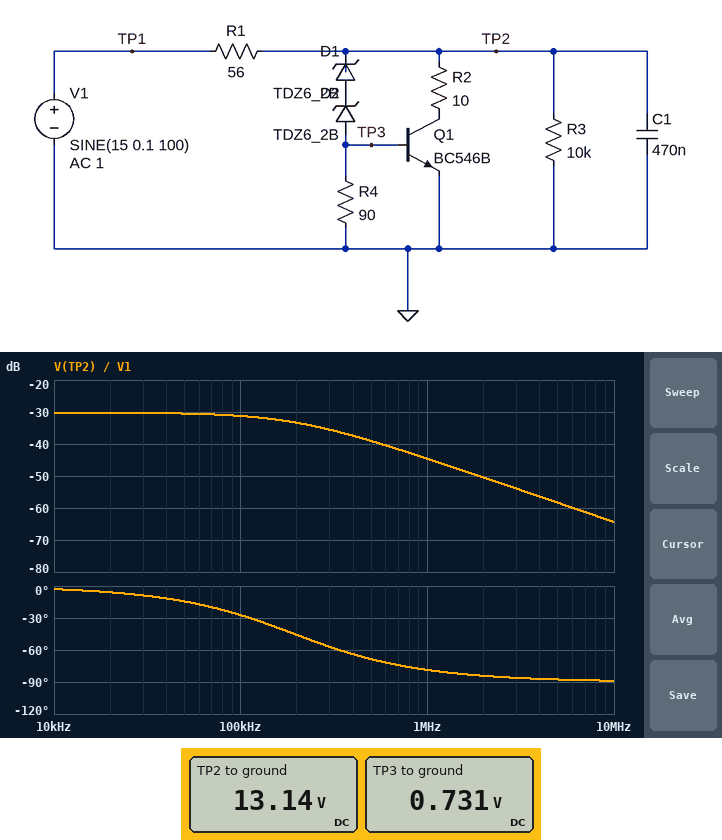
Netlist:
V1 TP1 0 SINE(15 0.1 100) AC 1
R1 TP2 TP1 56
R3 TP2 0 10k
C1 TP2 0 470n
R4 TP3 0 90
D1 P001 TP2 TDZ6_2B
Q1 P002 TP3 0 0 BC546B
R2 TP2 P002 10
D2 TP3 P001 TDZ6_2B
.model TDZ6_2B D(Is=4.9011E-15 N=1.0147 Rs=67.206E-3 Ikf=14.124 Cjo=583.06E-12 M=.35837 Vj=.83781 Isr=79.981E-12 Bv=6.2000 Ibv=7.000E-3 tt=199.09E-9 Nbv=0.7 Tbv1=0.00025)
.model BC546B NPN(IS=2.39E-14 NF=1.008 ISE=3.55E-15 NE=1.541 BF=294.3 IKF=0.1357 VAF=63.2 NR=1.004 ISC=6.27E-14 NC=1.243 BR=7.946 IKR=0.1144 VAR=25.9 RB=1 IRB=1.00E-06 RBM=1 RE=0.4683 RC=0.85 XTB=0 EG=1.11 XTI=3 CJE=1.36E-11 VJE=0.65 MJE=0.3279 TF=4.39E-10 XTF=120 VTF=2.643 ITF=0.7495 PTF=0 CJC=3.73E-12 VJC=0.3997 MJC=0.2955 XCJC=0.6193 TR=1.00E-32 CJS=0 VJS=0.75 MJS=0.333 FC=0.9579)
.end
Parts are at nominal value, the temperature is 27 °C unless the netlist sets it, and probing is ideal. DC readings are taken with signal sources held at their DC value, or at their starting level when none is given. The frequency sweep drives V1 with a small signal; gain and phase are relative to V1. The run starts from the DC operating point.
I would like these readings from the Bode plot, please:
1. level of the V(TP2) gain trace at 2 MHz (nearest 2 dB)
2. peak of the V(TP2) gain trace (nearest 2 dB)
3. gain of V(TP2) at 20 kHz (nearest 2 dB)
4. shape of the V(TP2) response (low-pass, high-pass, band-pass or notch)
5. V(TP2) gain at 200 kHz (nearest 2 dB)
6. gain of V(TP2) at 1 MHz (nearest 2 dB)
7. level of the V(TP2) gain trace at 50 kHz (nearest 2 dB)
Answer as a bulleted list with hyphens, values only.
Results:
- -50 dB
- -30 dB
- -30 dB
- low-pass
- -34 dB
- -44 dB
- -30 dB
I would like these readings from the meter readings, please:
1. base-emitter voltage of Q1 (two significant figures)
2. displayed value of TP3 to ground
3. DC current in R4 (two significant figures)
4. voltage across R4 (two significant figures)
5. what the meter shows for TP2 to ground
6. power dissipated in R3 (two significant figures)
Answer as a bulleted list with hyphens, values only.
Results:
- 730 mV
- 0.731 V
- 8.1 mA
- 730 mV
- 13.14 V
- 17 mW
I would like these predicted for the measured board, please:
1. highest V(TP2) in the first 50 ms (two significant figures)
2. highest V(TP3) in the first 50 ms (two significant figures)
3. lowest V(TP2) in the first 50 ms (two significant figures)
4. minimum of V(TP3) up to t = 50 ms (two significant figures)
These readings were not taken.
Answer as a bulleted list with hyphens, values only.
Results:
- 13 V
- 730 mV
- 13 V
- 730 mV
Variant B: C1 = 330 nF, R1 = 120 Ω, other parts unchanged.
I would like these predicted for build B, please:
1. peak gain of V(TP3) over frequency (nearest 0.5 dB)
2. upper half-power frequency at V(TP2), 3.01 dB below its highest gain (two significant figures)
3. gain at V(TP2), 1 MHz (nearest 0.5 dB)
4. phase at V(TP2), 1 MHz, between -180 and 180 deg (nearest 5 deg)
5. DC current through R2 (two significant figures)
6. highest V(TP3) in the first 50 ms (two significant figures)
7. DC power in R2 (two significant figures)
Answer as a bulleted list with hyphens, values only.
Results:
- -29.5 dB
- 110 kHz
- -48.0 dB
- -85 deg
- 6.9 mA
- 690 mV
- 480 µW
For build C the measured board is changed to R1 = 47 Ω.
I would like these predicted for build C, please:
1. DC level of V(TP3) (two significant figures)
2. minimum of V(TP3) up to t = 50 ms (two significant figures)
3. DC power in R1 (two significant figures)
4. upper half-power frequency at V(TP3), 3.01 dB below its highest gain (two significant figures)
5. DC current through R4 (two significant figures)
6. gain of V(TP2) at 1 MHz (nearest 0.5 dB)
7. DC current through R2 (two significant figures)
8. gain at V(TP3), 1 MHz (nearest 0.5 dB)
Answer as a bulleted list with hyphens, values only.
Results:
- 740 mV
- 740 mV
- 73 mW
- 220 kHz
- 8.2 mA
- -43.0 dB
- 30 mA
- -43.5 dB
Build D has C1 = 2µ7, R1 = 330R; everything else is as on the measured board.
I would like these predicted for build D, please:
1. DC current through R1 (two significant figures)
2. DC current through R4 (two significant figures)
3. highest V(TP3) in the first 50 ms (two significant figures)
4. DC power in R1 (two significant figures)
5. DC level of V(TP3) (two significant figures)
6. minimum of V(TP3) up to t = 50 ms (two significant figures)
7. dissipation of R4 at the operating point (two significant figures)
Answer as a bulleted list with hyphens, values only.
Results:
- 6.5 mA
- 5.2 mA
- 490 mV
- 14 mW
- 470 mV
- 450 mV
- 2.4 mW
